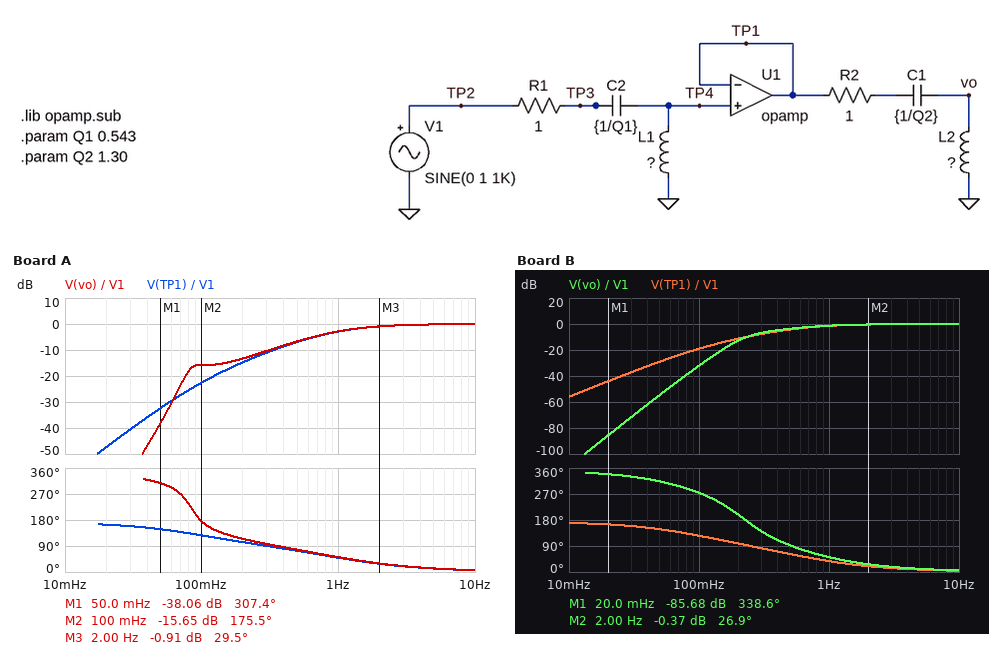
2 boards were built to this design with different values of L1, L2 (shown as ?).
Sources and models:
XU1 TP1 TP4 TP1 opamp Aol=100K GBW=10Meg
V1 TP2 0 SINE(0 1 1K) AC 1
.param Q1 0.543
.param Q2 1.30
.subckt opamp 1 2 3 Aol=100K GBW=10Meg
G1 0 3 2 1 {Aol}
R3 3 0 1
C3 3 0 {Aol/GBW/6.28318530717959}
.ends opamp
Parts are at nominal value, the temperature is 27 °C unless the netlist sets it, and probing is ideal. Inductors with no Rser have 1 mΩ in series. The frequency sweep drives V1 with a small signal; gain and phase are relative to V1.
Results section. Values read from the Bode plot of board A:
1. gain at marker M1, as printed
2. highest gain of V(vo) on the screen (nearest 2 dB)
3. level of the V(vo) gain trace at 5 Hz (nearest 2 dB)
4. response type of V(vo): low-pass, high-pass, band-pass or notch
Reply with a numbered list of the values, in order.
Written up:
1. -38.06 dB
2. 0 dB
3. 0 dB
4. high-pass
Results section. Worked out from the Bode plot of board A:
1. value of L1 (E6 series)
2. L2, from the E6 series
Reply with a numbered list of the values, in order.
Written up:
1. 150 mH
2. 4.7 H
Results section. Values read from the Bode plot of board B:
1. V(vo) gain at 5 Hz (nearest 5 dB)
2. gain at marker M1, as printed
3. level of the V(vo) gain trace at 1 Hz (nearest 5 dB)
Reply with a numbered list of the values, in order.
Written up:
1. 0 dB
2. -85.68 dB
3. 0 dB
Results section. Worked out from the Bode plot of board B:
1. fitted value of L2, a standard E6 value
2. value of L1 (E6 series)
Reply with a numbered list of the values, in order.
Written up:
1. 680 mH
2. 220 mH
